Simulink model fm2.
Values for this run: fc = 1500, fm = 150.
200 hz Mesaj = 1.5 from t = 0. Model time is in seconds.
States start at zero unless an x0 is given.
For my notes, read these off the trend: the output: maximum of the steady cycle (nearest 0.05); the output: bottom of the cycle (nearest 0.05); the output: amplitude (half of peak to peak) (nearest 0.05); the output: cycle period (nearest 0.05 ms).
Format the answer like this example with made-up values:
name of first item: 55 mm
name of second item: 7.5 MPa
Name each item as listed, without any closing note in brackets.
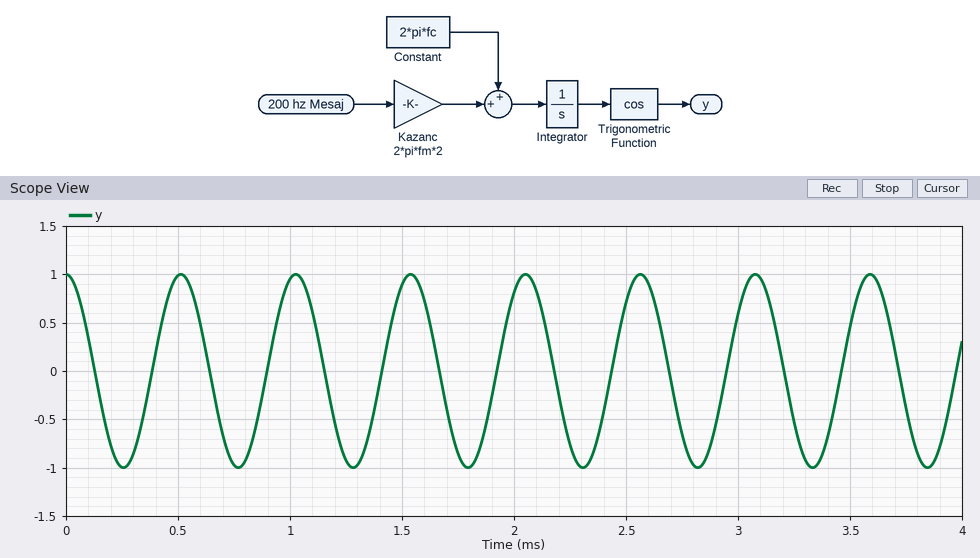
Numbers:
the output: maximum of the steady cycle: 1.00
the output: bottom of the cycle: -1.00
the output: amplitude (half of peak to peak): 1.00
the output: cycle period: 0.50 ms
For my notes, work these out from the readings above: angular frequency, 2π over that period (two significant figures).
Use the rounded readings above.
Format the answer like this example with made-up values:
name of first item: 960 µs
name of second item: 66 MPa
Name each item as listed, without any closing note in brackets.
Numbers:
angular frequency, 2π over that period: 13 rad/ms
